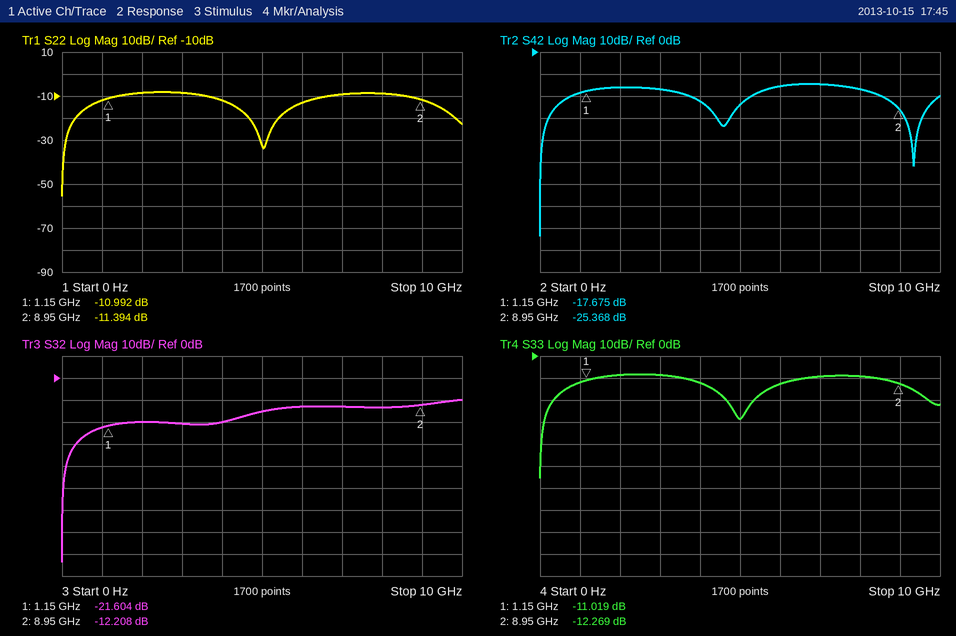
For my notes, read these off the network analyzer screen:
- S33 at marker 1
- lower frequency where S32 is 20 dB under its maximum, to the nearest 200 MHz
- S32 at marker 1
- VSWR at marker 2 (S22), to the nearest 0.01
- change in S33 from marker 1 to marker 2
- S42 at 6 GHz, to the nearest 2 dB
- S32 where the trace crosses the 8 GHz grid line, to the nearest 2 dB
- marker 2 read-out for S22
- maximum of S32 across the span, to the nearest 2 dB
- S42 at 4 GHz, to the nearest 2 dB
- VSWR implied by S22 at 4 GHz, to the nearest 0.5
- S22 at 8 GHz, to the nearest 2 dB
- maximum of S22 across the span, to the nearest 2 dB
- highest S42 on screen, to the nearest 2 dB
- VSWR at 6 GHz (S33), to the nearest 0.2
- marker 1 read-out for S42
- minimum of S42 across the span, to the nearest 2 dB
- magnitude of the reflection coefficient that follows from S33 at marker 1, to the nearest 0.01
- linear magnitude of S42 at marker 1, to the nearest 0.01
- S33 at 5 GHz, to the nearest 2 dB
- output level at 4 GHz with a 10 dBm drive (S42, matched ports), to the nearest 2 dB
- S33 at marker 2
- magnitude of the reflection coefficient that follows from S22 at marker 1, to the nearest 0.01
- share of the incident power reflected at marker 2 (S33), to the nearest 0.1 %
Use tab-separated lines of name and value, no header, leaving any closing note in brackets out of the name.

S33 at marker 1	-11.019 dB
lower frequency where S32 is 20 dB under its maximum, to the nearest 200 MHz	400 MHz
S32 at marker 1	-21.604 dB
VSWR at marker 2 (S22), to the nearest 0.01	1.74
change in S33 from marker 1 to marker 2	-1.250 dB
S42 at 6 GHz, to the nearest 2 dB	-16 dB
S32 where the trace crosses the 8 GHz grid line, to the nearest 2 dB	-14 dB
marker 2 read-out for S22	-11.394 dB
maximum of S32 across the span, to the nearest 2 dB	-10 dB
S42 at 4 GHz, to the nearest 2 dB	-22 dB
VSWR implied by S22 at 4 GHz, to the nearest 0.5	1.5
S22 at 8 GHz, to the nearest 2 dB	-8 dB
maximum of S22 across the span, to the nearest 2 dB	-8 dB
highest S42 on screen, to the nearest 2 dB	-14 dB
VSWR at 6 GHz (S33), to the nearest 0.2	1.6
marker 1 read-out for S42	-17.675 dB
minimum of S42 across the span, to the nearest 2 dB	-84 dB
magnitude of the reflection coefficient that follows from S33 at marker 1, to the nearest 0.01	0.28
linear magnitude of S42 at marker 1, to the nearest 0.01	0.13
S33 at 5 GHz, to the nearest 2 dB	-28 dB
output level at 4 GHz with a 10 dBm drive (S42, matched ports), to the nearest 2 dB	-12 dBm
S33 at marker 2	-12.269 dB
magnitude of the reflection coefficient that follows from S22 at marker 1, to the nearest 0.01	0.28
share of the incident power reflected at marker 2 (S33), to the nearest 0.1 %	5.9 %
